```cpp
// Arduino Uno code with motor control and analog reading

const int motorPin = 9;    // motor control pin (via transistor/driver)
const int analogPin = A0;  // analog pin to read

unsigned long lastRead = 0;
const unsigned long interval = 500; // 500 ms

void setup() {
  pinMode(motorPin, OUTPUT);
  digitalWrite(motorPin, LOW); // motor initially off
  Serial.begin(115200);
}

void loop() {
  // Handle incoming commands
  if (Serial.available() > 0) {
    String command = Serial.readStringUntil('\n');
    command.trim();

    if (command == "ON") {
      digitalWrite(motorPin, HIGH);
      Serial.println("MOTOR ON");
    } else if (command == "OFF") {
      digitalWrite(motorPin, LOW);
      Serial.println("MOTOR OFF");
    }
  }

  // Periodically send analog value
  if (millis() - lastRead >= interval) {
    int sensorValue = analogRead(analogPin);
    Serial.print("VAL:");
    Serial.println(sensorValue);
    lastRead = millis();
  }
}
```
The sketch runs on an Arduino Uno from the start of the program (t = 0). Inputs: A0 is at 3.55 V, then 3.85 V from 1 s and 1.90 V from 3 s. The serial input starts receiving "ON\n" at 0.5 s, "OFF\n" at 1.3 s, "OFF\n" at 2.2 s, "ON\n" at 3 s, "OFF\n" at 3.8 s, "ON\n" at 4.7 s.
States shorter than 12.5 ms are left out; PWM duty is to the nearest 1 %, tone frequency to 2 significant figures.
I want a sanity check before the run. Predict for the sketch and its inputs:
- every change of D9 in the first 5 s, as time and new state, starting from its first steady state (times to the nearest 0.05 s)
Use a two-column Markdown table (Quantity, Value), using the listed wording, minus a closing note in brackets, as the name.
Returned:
| Quantity | Value |
|---|---|
| every change of D9 in the first 5 s, as time and new state, starting from its first steady state | 0 s low; 0.5 s high; 1.3 s low; 3 s high; 3.8 s low; 4.7 s high |
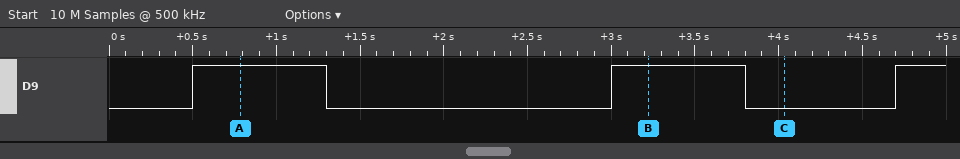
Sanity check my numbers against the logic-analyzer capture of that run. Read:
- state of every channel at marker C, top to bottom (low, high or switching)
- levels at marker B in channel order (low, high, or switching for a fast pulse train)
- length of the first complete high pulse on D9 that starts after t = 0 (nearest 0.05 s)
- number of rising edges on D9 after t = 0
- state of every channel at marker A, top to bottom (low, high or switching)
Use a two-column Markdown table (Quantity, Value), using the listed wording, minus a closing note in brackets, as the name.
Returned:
| Quantity | Value |
|---|---|
| state of every channel at marker C, top to bottom | D9 low |
| levels at marker B in channel order | D9 high |
| length of the first complete high pulse on D9 that starts after t = 0 | 0.80 s |
| number of rising edges on D9 after t = 0 | 3 |
| state of every channel at marker A, top to bottom | D9 high |
